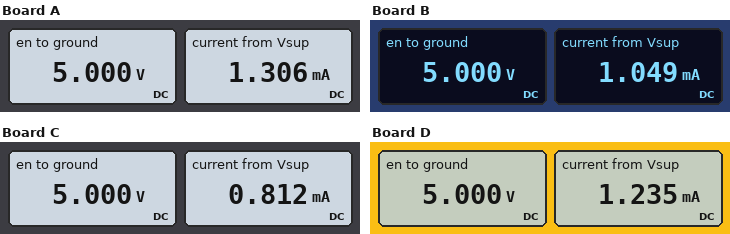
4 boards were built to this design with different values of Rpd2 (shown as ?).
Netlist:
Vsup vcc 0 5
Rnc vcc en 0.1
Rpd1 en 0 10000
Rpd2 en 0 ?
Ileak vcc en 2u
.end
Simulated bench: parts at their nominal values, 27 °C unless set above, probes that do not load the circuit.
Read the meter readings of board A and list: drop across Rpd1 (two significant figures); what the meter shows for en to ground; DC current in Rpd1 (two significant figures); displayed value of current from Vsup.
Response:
5.0 V
5.000 V
500 µA
1.306 mA
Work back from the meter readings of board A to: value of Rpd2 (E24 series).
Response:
6.2 kΩ
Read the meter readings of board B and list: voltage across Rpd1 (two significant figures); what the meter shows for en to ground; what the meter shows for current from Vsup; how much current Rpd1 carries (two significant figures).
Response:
5.0 V
5.000 V
1.049 mA
500 µA
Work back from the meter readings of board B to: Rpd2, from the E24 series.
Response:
9.1 kΩ
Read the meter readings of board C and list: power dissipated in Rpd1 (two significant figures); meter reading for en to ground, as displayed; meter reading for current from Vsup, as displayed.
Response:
2.5 mW
5.000 V
0.812 mA
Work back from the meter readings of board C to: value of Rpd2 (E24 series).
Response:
16 kΩ
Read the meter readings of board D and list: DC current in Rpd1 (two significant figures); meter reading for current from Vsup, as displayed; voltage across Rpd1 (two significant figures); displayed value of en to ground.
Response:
500 µA
1.235 mA
5.0 V
5.000 V
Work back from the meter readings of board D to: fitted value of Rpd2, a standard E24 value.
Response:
6.8 kΩ
